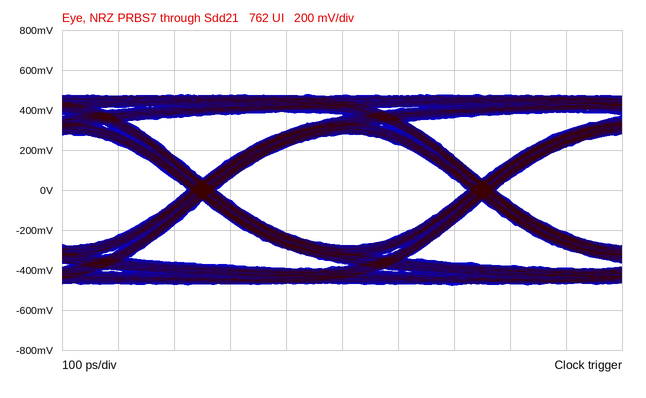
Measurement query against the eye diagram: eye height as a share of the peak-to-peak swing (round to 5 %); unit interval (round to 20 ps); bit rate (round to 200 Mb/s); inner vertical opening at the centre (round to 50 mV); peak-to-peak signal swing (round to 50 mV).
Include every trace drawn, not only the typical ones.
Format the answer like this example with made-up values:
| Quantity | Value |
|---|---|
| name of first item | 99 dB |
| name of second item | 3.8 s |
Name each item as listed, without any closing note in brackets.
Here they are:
| Quantity | Value |
|---|---|
| eye height as a share of the peak-to-peak swing | 60 % |
| unit interval | 500 ps |
| bit rate | 2.0 Gb/s |
| inner vertical opening at the centre | 550 mV |
| peak-to-peak signal swing | 950 mV |
